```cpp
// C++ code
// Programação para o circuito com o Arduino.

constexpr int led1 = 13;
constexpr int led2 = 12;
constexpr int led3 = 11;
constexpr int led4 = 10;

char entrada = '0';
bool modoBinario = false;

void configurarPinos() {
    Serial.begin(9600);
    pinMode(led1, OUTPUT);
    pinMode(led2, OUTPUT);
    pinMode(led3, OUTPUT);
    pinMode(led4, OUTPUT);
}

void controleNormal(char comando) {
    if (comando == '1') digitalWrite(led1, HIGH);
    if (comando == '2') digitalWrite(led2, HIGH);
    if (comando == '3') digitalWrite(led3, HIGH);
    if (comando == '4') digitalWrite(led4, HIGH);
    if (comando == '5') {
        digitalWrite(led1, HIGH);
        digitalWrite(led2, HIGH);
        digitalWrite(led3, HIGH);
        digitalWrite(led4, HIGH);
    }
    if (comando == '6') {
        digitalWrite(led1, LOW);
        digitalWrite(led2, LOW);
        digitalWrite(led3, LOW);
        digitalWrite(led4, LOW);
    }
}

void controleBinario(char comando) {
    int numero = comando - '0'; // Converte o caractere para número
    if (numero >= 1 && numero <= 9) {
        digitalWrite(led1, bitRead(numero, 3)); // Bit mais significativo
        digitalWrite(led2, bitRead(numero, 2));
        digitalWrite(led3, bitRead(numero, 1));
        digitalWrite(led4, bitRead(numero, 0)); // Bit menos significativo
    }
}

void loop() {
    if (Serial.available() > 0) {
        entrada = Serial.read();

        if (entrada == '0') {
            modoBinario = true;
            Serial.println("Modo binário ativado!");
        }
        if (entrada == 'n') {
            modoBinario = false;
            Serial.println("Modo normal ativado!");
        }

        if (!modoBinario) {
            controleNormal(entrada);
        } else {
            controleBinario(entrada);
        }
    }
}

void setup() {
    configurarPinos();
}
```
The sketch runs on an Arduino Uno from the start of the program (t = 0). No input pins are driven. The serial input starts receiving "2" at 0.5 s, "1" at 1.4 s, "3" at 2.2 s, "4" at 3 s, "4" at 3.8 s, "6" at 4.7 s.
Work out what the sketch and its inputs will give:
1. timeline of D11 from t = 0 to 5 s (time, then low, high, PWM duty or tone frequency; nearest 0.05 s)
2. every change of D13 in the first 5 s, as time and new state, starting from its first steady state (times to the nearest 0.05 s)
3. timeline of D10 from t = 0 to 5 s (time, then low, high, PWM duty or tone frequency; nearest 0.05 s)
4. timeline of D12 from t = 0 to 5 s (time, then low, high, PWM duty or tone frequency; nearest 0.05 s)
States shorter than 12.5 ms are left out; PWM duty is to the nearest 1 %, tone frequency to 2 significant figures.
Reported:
0 s low; 2.2 s high; 4.7 s low
0 s low; 1.4 s high; 4.7 s low
0 s low; 3 s high; 4.7 s low
0 s low; 0.5 s high; 4.7 s low
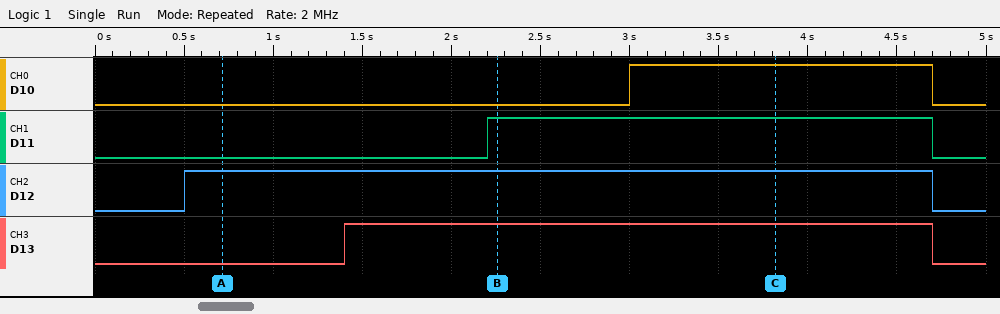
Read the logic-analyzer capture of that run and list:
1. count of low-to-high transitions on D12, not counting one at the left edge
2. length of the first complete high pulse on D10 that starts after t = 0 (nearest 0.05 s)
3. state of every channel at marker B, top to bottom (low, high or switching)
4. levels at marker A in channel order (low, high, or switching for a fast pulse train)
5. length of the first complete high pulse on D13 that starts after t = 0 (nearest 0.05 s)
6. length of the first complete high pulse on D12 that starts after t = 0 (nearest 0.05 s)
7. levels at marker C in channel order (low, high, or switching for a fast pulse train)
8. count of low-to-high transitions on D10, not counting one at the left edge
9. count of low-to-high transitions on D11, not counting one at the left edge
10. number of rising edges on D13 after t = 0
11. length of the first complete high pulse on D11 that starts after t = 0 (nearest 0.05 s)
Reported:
1
1.70 s
D10 low, D11 high, D12 high, D13 high
D10 low, D11 low, D12 high, D13 low
3.30 s
4.20 s
D10 high, D11 high, D12 high, D13 high
1
1
1
2.50 s
